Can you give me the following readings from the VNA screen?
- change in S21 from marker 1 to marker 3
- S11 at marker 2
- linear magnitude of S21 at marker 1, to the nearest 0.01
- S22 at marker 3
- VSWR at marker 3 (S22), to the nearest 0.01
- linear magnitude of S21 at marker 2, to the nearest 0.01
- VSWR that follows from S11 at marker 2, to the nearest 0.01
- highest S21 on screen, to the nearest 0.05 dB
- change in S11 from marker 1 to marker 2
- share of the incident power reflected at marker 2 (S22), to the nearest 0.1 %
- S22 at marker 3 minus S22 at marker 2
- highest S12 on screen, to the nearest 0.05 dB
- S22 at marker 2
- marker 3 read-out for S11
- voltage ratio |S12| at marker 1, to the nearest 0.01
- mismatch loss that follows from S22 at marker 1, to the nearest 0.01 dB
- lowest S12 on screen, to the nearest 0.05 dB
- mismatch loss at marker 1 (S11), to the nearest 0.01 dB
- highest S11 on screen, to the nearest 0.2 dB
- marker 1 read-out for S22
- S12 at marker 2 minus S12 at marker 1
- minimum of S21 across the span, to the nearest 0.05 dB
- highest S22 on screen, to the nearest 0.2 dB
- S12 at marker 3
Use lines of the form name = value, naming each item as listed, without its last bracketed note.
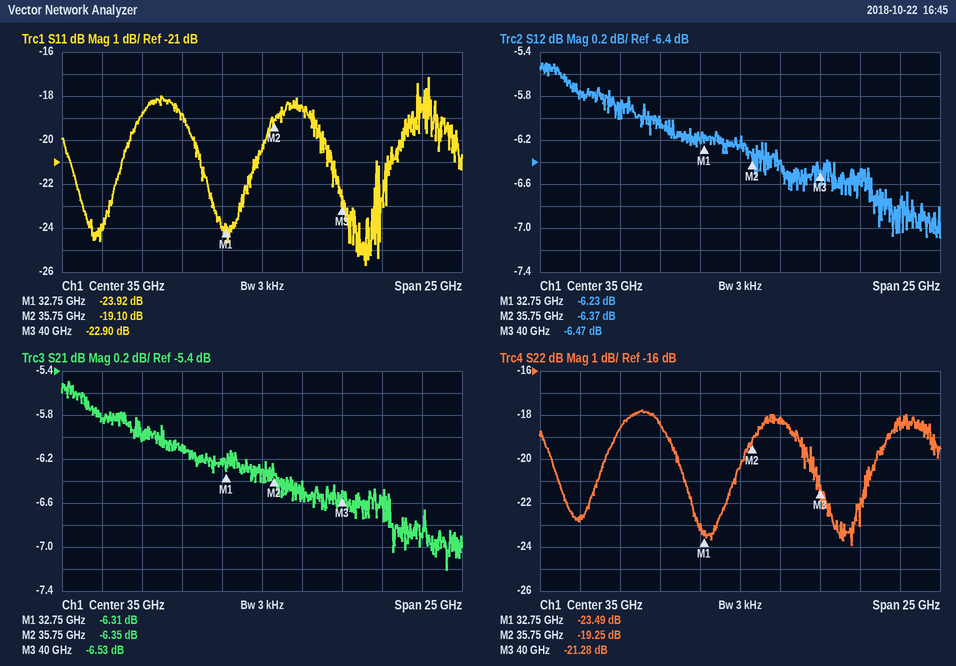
change in S21 from marker 1 to marker 3 = -0.22 dB
S11 at marker 2 = -19.10 dB
linear magnitude of S21 at marker 1, to the nearest 0.01 = 0.48
S22 at marker 3 = -21.28 dB
VSWR at marker 3 (S22), to the nearest 0.01 = 1.19
linear magnitude of S21 at marker 2, to the nearest 0.01 = 0.48
VSWR that follows from S11 at marker 2, to the nearest 0.01 = 1.25
highest S21 on screen, to the nearest 0.05 dB = -5.50 dB
change in S11 from marker 1 to marker 2 = 4.82 dB
share of the incident power reflected at marker 2 (S22), to the nearest 0.1 % = 1.2 %
S22 at marker 3 minus S22 at marker 2 = -2.03 dB
highest S12 on screen, to the nearest 0.05 dB = -5.50 dB
S22 at marker 2 = -19.25 dB
marker 3 read-out for S11 = -22.90 dB
voltage ratio |S12| at marker 1, to the nearest 0.01 = 0.49
mismatch loss that follows from S22 at marker 1, to the nearest 0.01 dB = 0.02 dB
lowest S12 on screen, to the nearest 0.05 dB = -7.10 dB
mismatch loss at marker 1 (S11), to the nearest 0.01 dB = 0.02 dB
highest S11 on screen, to the nearest 0.2 dB = -17.2 dB
marker 1 read-out for S22 = -23.49 dB
S12 at marker 2 minus S12 at marker 1 = -0.14 dB
minimum of S21 across the span, to the nearest 0.05 dB = -7.20 dB
highest S22 on screen, to the nearest 0.2 dB = -17.8 dB
S12 at marker 3 = -6.47 dB
